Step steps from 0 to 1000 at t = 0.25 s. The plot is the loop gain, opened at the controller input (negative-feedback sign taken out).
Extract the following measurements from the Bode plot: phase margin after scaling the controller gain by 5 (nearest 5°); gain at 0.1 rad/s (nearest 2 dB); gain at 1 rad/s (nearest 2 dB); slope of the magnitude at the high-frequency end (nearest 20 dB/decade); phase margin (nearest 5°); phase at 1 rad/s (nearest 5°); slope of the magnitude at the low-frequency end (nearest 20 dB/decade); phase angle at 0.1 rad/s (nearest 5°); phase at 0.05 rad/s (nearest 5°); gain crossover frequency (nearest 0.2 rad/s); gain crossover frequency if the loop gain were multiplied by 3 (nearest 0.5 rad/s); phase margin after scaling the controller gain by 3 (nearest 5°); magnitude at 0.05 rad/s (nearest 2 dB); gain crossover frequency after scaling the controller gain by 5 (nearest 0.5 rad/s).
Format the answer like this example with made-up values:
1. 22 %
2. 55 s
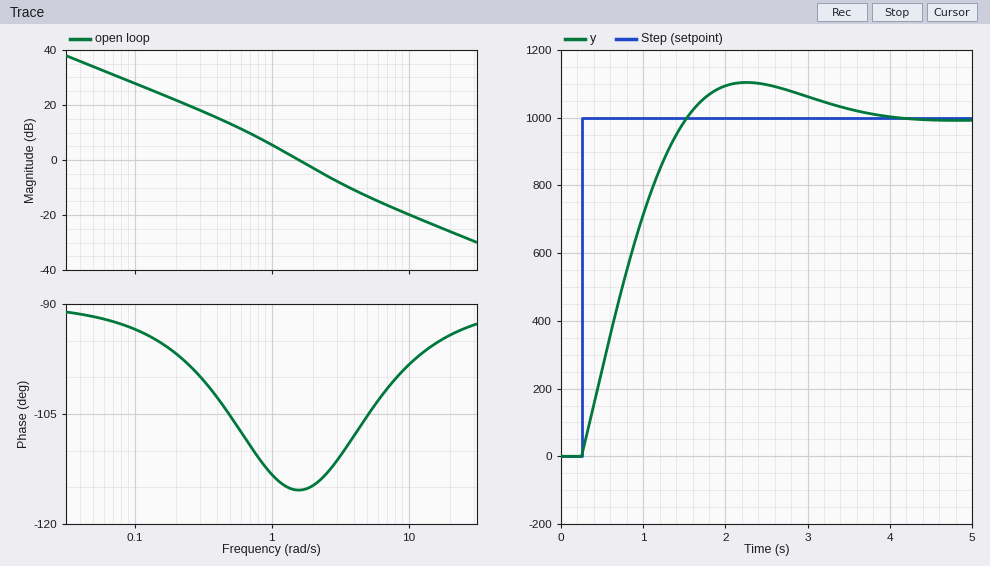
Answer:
1. 75°
2. 28 dB
3. 6 dB
4. -20 dB/decade
5. 65°
6. -115°
7. -20 dB/decade
8. -95°
9. -90°
10. 1.6 rad/s
11. 3.5 rad/s
12. 70°
13. 34 dB
14. 5.5 rad/s
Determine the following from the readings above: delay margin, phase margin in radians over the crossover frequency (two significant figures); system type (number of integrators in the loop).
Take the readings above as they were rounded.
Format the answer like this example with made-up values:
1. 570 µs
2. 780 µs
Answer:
1. 0.71 s
2. 1
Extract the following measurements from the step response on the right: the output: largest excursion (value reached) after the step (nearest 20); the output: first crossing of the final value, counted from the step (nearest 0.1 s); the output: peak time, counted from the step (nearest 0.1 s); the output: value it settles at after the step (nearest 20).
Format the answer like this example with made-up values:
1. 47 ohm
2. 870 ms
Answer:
1. 1100
2. 1.3 s
3. 2.0 s
4. 1000
